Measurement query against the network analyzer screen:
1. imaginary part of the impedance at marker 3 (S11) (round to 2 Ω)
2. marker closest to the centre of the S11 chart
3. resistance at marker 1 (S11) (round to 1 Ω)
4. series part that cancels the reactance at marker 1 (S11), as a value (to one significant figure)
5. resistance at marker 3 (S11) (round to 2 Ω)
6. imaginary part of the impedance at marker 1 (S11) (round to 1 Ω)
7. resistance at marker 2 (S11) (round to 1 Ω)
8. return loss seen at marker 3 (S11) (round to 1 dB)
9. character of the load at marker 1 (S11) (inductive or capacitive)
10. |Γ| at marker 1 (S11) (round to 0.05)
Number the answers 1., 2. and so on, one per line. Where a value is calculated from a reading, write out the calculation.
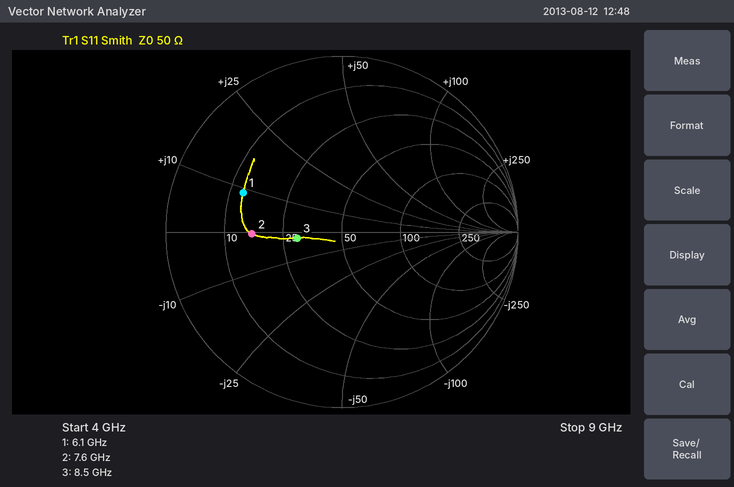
1. -2 Ω
2. marker 3
3. 13 Ω
4. C = 1/(2π × 6.1 GHz × 9 Ω) ≈ 3 pF
5. 30 Ω
6. +9 Ω
7. 16 Ω
8. 12 dB
9. inductive
10. 0.60
